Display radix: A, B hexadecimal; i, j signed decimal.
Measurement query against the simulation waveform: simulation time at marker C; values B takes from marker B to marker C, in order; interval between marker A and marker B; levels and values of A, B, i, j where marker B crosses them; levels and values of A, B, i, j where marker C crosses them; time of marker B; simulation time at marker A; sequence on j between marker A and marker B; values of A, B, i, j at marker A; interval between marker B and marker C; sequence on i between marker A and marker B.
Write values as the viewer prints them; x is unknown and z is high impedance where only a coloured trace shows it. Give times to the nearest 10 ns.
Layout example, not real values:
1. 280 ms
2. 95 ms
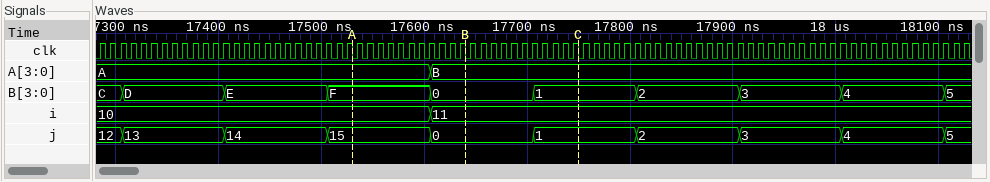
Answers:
1. 17750 ns
2. 0, 1
3. 110 ns
4. A=B, B=0, i=11, j=0
5. A=B, B=1, i=11, j=1
6. 17640 ns
7. 17530 ns
8. 15, 0
9. A=A, B=F, i=10, j=15
10. 110 ns
11. 10, 11
